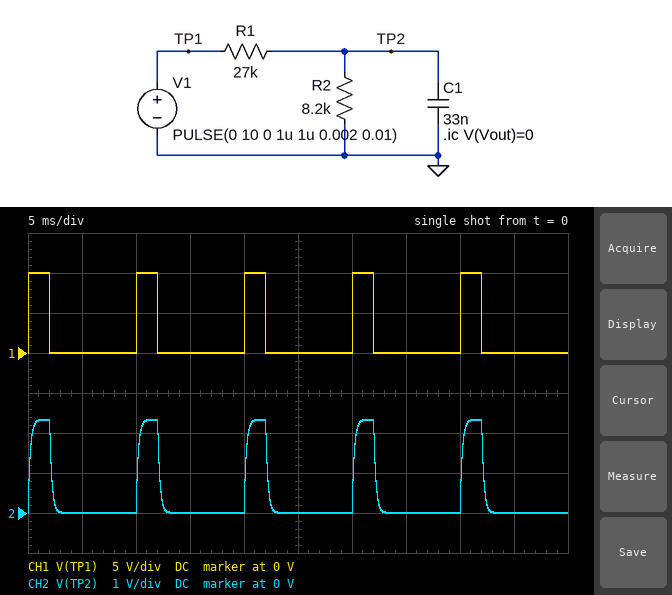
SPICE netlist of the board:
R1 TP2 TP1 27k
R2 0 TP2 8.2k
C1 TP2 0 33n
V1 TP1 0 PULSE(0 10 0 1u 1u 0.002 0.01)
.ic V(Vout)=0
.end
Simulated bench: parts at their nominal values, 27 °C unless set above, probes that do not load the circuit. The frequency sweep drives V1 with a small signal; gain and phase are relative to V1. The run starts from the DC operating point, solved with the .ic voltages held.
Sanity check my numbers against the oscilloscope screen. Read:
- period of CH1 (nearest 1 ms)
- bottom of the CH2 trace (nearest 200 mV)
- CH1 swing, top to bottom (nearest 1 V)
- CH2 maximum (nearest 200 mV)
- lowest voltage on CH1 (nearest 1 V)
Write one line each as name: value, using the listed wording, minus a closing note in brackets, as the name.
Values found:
period of CH1: 10 ms
bottom of the CH2 trace: 0 V
CH1 swing, top to bottom: 10 V
CH2 maximum: 2.4 V
lowest voltage on CH1: 0 V
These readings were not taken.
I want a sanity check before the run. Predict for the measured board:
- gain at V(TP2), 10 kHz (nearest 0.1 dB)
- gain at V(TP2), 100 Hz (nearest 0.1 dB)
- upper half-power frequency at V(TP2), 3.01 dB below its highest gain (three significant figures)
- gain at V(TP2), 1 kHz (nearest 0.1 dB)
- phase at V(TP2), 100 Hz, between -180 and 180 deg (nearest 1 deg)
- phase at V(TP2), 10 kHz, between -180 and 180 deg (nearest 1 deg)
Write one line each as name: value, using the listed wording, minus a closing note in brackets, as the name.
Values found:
gain at V(TP2), 10 kHz: -35.0 dB
gain at V(TP2), 100 Hz: -12.7 dB
upper half-power frequency at V(TP2), 3.01 dB below its highest gain: 767 Hz
gain at V(TP2), 1 kHz: -17.0 dB
phase at V(TP2), 100 Hz, between -180 and 180 deg: -7 deg
phase at V(TP2), 10 kHz, between -180 and 180 deg: -86 deg
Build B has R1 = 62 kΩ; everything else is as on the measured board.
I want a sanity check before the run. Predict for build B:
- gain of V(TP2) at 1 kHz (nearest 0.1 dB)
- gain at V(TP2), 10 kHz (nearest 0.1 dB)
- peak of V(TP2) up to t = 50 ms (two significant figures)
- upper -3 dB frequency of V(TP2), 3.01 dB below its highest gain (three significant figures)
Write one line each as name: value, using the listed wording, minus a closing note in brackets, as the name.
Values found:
gain of V(TP2) at 1 kHz: -23.8 dB
gain at V(TP2), 10 kHz: -42.2 dB
peak of V(TP2) up to t = 50 ms: 1.2 V
upper -3 dB frequency of V(TP2), 3.01 dB below its highest gain: 666 Hz
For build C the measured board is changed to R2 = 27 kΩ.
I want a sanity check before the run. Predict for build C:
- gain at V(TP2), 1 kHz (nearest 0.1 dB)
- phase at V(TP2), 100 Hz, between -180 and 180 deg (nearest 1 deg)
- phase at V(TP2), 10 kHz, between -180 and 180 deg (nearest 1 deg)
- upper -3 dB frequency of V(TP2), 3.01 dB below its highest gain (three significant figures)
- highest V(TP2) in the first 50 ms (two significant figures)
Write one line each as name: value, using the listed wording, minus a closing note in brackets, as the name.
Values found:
gain at V(TP2), 1 kHz: -15.5 dB
phase at V(TP2), 100 Hz, between -180 and 180 deg: -16 deg
phase at V(TP2), 10 kHz, between -180 and 180 deg: -88 deg
upper -3 dB frequency of V(TP2), 3.01 dB below its highest gain: 357 Hz
highest V(TP2) in the first 50 ms: 4.9 V
